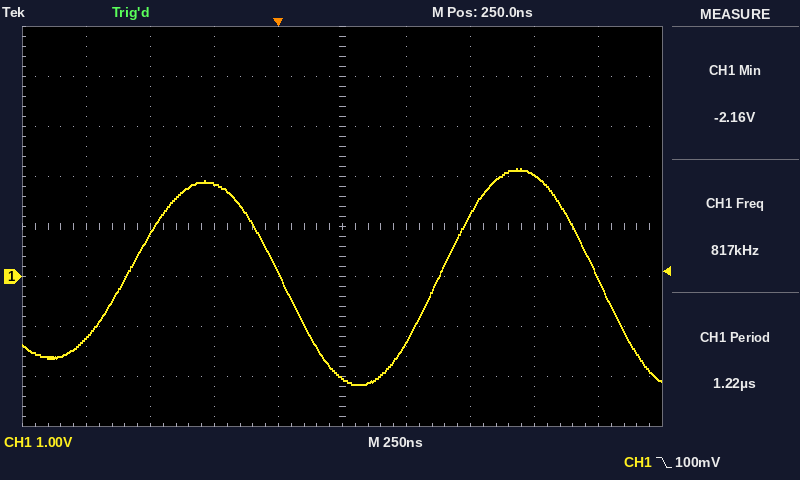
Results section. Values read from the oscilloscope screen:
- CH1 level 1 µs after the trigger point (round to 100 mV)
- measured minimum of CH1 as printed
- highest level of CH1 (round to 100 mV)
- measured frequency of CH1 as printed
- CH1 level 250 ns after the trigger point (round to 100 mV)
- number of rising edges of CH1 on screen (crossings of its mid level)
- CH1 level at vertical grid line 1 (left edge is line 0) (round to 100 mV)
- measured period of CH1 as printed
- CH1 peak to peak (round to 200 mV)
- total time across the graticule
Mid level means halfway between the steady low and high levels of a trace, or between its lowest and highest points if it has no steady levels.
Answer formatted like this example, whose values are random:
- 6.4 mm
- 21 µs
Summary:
- 2.0 V
- -2.16 V
- 2.2 V
- 817 kHz
- -2.0 V
- 2
- -1.2 V
- 1.22 µs
- 4.4 V
- 2.5 µs
